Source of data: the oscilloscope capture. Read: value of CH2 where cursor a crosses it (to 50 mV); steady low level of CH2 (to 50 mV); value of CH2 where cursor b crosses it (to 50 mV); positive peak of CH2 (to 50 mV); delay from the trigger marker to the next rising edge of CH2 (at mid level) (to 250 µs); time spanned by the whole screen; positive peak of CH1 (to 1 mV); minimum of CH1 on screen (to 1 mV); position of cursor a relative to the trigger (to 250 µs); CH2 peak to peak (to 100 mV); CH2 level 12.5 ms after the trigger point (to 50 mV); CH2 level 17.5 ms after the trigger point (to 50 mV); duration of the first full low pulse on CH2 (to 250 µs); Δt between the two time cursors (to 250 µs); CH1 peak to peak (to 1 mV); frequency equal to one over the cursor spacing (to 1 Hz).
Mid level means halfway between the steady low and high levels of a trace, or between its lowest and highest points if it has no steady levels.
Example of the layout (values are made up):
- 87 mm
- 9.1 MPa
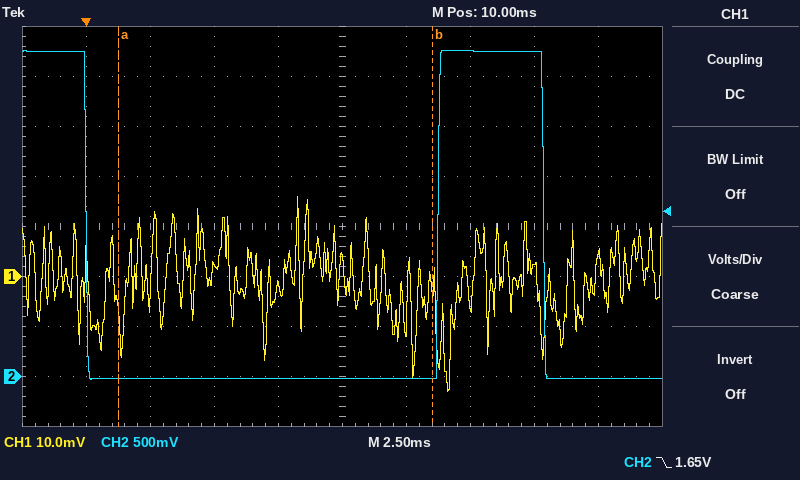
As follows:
- 0 mV
- 0 mV
- 0 mV
- 3.25 V
- 13.75 ms
- 25 ms
- 16 mV
- -23 mV
- +1.25 ms
- 3.30 V
- 0 mV
- 3.25 V
- 13.75 ms
- 12.25 ms
- 39 mV
- 82 Hz
